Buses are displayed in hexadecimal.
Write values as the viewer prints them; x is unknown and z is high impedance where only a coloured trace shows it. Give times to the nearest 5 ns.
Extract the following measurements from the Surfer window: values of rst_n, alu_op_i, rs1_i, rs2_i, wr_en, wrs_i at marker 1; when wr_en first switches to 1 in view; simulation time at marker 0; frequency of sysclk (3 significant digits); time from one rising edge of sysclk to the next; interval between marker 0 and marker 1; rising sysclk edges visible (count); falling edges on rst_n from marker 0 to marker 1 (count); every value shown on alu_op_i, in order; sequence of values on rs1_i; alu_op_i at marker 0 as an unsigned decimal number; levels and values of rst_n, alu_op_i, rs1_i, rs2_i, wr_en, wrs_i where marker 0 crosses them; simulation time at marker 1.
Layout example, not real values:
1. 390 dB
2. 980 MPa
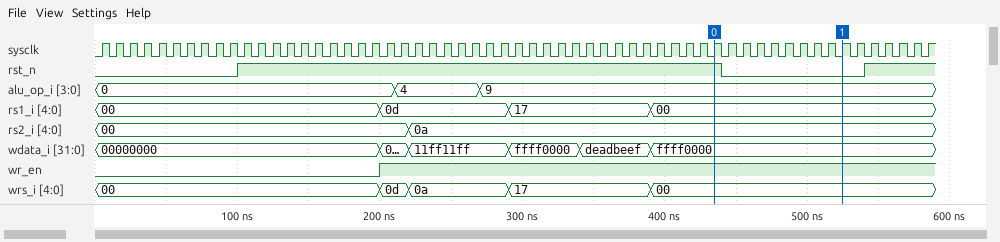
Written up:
1. rst_n=0, alu_op_i=9, rs1_i=00, rs2_i=0a, wr_en=1, wrs_i=00
2. 200 ns
3. 435 ns
4. 100 MHz
5. 10 ns
6. 90 ns
7. 59
8. 1
9. 0, 4, 9
10. 00, 0d, 17, 00
11. 9
12. rst_n=1, alu_op_i=9, rs1_i=00, rs2_i=0a, wr_en=1, wrs_i=00
13. 525 ns
